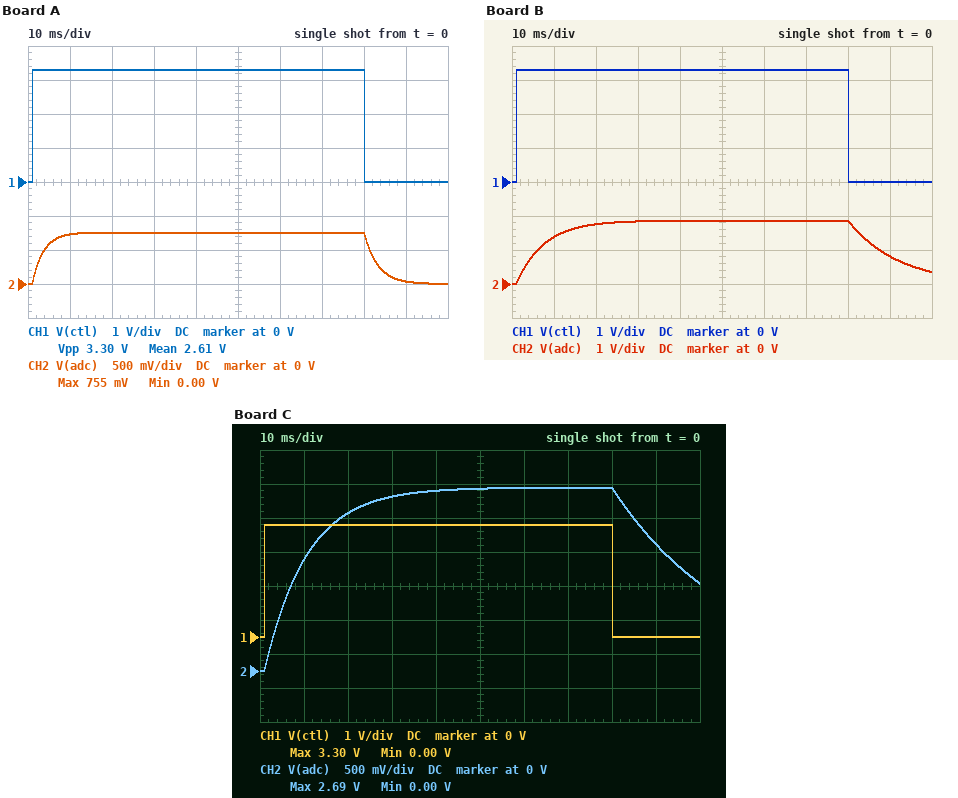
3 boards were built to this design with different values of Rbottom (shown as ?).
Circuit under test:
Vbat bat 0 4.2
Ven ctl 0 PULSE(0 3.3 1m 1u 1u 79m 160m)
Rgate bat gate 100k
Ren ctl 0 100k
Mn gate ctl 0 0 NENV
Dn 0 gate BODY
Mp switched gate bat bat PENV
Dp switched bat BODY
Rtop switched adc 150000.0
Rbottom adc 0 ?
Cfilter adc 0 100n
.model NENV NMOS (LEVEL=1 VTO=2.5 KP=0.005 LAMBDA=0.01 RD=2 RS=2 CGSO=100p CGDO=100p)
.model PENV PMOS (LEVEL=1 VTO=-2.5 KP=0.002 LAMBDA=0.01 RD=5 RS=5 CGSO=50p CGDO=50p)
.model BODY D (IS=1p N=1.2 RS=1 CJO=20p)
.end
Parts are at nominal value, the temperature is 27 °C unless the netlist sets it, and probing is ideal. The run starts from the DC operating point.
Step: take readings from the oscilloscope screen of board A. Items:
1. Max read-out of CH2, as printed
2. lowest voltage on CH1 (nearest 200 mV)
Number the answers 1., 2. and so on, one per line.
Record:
1. 755 mV
2. 0 V
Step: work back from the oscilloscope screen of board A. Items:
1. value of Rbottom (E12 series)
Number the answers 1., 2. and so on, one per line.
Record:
1. 33 kΩ
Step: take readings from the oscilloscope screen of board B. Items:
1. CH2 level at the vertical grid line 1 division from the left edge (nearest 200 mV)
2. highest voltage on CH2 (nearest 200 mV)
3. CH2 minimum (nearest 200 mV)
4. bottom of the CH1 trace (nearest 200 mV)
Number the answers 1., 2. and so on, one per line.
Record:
1. 1.4 V
2. 1.8 V
3. 0 V
4. 0 V
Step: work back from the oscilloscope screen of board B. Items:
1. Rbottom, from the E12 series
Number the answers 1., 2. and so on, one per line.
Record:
1. 120 kΩ
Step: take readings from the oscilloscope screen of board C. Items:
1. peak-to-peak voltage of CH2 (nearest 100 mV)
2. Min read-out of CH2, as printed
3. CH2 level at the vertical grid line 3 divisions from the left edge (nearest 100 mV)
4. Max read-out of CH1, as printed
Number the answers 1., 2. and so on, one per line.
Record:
1. 2.7 V
2. 0.00 V
3. 2.6 V
4. 3.30 V
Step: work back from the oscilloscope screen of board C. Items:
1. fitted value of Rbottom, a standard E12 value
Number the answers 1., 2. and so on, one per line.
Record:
1. 270 kΩ
